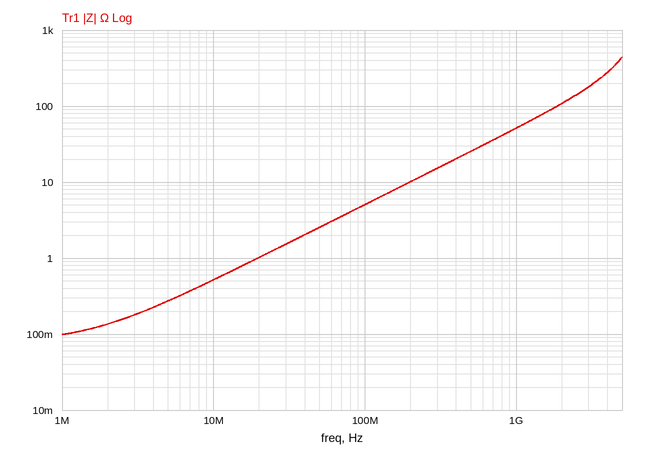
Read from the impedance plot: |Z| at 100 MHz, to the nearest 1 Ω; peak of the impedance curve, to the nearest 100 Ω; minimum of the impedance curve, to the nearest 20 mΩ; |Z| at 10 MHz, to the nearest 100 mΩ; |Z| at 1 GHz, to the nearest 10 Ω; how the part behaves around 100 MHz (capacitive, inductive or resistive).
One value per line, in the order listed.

5 Ω
400 Ω
100 mΩ
500 mΩ
50 Ω
inductive
